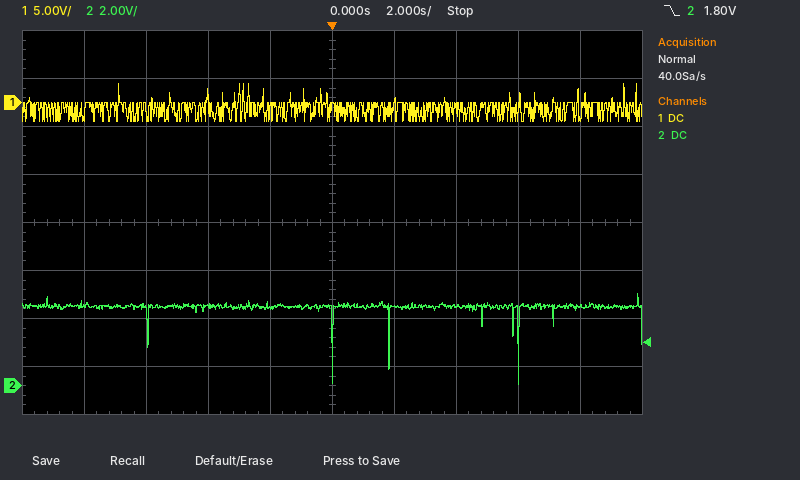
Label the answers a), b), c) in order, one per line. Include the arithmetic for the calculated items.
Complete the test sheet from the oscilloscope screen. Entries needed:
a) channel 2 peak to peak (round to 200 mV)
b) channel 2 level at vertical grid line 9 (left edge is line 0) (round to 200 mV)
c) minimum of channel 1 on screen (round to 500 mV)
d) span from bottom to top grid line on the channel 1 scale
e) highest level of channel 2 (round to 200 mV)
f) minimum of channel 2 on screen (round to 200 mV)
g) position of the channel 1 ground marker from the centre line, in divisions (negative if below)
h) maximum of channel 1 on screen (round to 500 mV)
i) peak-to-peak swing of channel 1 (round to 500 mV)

a) 3.8 V − (0.0 V) = 3.8 V
b) 3.4 V
c) -2.0 V
d) 40 V
e) 3.8 V
f) 0.0 V
g) +2.5 div
h) 2.0 V
i) 2.0 V − (-2.0 V) = 4.0 V
